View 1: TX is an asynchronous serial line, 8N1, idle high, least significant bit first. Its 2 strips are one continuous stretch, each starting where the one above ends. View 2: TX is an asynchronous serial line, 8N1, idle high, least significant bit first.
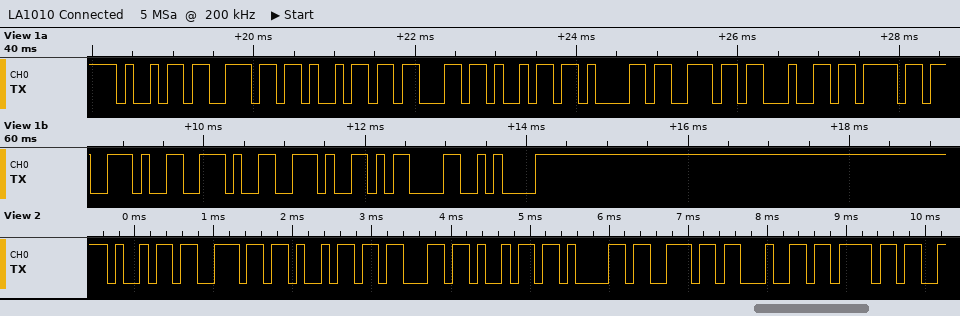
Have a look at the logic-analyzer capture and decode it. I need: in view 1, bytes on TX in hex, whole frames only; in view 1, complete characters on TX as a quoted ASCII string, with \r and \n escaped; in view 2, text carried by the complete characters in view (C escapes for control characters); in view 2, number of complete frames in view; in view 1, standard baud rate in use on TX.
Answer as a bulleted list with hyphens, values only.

- 69 6E 69 63 69 61 6E 64 6F 2E 2E 2E 0D 0A
- "iniciando...\r\n"
- "iniciando"
- 9
- 9600 baud
